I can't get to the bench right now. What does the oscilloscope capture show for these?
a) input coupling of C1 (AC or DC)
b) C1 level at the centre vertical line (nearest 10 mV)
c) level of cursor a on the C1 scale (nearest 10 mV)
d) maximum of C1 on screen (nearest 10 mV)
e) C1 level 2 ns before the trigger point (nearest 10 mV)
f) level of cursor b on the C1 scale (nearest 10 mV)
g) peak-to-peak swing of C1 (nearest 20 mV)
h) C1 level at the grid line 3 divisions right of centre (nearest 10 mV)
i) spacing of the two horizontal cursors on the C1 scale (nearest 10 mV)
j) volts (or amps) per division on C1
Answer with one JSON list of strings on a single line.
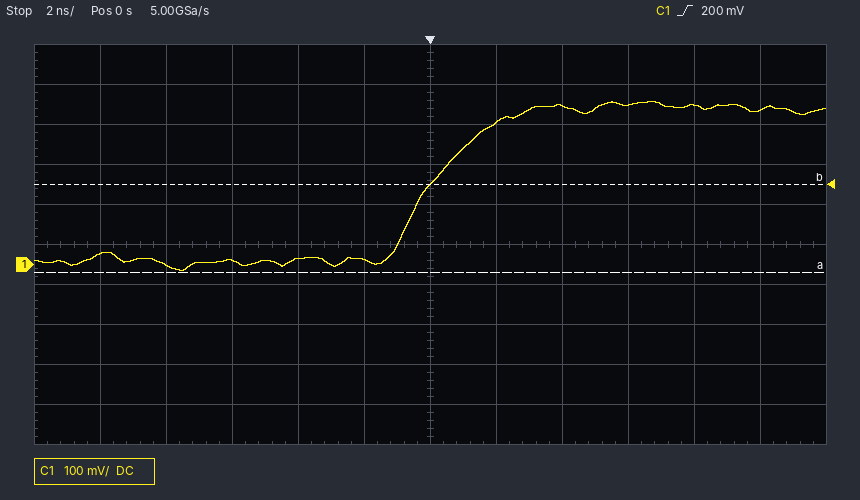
["DC", "200 mV", "-20 mV", "410 mV", "10 mV", "200 mV", "420 mV", "400 mV", "220 mV", "100 mV"]
